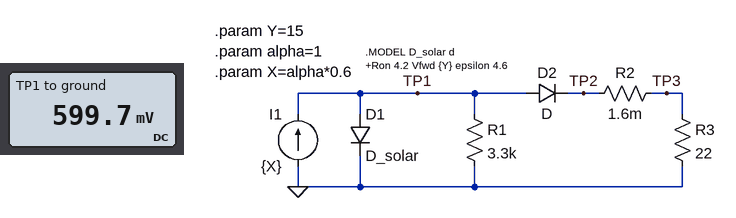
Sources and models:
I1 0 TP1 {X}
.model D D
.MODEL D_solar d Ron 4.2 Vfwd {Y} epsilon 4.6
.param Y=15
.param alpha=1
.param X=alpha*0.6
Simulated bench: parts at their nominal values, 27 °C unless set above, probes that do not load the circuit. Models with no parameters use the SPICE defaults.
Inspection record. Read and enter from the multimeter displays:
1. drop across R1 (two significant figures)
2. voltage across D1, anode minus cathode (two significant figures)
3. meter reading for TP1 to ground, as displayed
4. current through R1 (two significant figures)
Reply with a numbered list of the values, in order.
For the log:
1. 600 mV
2. 600 mV
3. 599.7 mV
4. 180 µA
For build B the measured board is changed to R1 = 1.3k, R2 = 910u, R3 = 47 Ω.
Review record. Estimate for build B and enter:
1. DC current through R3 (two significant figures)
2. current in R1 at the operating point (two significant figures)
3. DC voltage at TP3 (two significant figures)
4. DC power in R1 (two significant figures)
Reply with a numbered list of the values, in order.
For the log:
1. 97 µA
2. 460 µA
3. 4.6 mV
4. 280 µW
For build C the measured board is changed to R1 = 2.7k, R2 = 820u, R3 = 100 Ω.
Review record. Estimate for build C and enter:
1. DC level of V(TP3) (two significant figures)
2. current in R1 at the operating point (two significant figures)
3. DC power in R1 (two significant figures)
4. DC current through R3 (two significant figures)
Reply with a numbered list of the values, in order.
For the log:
1. 8.5 mV
2. 220 µA
3. 130 µW
4. 85 µA
